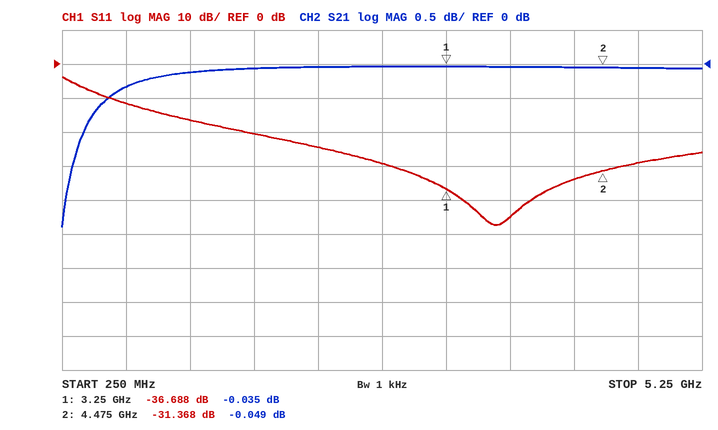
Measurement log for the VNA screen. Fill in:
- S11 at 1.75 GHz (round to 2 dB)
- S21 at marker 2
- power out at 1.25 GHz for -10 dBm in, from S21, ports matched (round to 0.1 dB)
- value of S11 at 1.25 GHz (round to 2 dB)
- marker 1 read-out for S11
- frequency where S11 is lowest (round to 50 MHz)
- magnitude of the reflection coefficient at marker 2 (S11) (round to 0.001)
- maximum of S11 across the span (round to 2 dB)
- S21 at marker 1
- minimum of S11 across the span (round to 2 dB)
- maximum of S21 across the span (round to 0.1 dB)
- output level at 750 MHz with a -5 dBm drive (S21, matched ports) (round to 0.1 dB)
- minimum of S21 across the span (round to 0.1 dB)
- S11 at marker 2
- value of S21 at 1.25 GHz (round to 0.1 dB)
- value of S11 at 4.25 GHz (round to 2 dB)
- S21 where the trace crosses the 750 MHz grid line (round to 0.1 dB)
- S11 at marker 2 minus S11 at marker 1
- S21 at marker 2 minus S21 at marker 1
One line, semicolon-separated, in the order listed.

-20 dB; -0.049 dB; -10.1 dBm; -16 dB; -36.688 dB; 3.65 GHz; 0.027; -4 dB; -0.035 dB; -48 dB; 0.0 dB; -5.3 dBm; -2.4 dB; -31.368 dB; -0.1 dB; -34 dB; -0.3 dB; 5.320 dB; -0.014 dB
